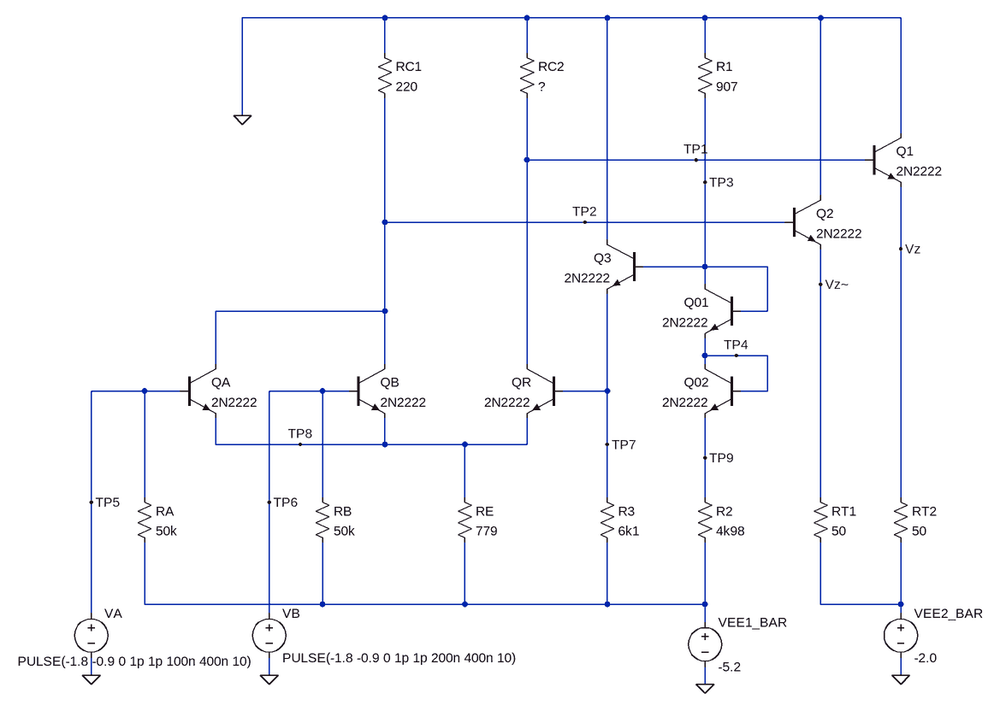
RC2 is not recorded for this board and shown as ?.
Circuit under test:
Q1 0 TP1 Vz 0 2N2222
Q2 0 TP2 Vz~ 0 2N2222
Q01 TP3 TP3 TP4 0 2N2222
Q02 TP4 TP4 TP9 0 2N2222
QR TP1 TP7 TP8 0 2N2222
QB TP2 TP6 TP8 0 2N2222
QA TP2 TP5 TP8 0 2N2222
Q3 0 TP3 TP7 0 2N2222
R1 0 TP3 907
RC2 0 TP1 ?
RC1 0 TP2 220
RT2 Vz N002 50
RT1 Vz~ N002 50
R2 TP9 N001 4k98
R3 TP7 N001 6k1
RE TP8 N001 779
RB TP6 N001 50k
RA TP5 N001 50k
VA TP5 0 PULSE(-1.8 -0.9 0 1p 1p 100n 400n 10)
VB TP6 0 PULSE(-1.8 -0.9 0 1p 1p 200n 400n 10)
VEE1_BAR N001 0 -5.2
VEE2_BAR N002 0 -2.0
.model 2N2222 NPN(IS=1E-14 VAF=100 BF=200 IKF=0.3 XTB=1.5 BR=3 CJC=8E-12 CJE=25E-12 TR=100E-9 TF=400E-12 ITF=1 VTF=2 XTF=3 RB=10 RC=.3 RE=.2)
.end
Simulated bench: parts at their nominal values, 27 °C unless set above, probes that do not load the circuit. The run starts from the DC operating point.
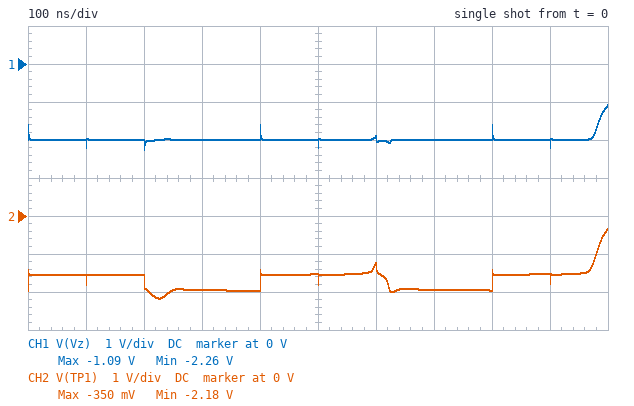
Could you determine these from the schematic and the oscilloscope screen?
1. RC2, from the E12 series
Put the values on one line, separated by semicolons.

680 Ω
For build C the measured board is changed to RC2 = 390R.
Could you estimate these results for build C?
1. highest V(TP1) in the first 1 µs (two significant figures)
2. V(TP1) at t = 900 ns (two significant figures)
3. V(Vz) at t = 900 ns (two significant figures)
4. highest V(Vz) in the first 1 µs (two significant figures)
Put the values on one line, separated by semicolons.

-41 mV; -51 mV; -800 mV; -790 mV
